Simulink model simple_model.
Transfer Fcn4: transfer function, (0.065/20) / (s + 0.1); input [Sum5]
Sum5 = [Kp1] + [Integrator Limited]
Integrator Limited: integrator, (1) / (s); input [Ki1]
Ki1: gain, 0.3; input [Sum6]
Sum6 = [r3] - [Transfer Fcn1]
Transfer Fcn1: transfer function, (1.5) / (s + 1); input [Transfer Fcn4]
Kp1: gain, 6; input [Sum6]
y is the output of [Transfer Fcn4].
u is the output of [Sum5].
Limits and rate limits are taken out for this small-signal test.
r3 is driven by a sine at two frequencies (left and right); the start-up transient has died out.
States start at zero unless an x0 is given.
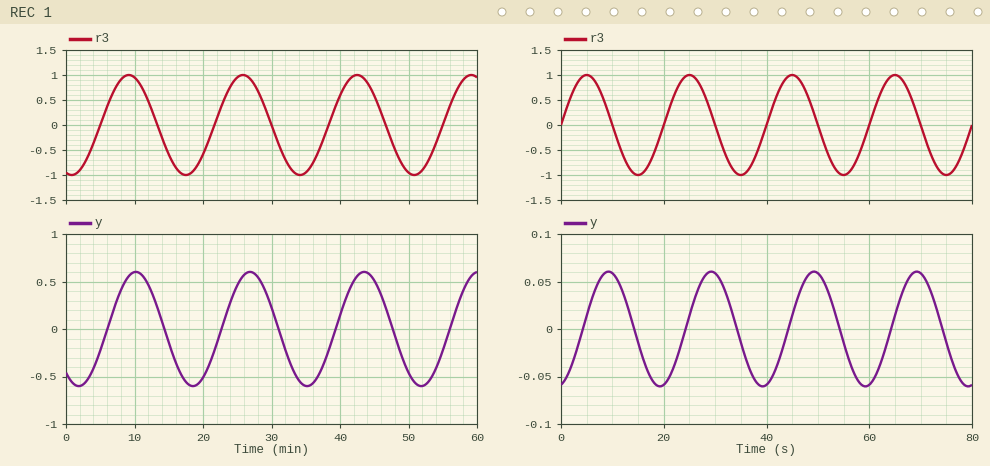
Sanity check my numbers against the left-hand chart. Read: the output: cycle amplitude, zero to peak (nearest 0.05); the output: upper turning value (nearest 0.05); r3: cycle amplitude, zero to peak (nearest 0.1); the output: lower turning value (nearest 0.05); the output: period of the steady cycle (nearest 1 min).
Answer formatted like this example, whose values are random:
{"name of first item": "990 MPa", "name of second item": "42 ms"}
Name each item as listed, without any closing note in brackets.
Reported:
{"the output: cycle amplitude, zero to peak": "0.60", "the output: upper turning value": "0.60", "r3: cycle amplitude, zero to peak": "1.0", "the output: lower turning value": "-0.60", "the output: period of the steady cycle": "17 min"}
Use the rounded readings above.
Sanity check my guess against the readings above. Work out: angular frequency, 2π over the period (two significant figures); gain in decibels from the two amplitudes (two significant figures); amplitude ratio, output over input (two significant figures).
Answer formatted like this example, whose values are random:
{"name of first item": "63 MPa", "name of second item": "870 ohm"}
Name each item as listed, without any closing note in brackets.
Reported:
{"angular frequency, 2π over the period": "0.37 rad/min", "gain in decibels from the two amplitudes": "-4.4 dB", "amplitude ratio, output over input": "0.60"}
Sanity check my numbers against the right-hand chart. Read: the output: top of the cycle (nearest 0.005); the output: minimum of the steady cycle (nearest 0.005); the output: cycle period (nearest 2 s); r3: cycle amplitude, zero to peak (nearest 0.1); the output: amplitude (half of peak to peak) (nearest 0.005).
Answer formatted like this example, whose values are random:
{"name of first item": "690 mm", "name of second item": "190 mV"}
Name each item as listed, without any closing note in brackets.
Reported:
{"the output: top of the cycle": "0.060", "the output: minimum of the steady cycle": "-0.060", "the output: cycle period": "20 s", "r3: cycle amplitude, zero to peak": "1.0", "the output: amplitude (half of peak to peak)": "0.060"}
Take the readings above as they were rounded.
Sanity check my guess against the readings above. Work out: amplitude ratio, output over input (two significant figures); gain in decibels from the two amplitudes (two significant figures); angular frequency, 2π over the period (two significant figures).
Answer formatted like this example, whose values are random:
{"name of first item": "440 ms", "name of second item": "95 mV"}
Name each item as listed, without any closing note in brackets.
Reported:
{"amplitude ratio, output over input": "0.060", "gain in decibels from the two amplitudes": "-24 dB", "angular frequency, 2π over the period": "0.31 rad/s"}
